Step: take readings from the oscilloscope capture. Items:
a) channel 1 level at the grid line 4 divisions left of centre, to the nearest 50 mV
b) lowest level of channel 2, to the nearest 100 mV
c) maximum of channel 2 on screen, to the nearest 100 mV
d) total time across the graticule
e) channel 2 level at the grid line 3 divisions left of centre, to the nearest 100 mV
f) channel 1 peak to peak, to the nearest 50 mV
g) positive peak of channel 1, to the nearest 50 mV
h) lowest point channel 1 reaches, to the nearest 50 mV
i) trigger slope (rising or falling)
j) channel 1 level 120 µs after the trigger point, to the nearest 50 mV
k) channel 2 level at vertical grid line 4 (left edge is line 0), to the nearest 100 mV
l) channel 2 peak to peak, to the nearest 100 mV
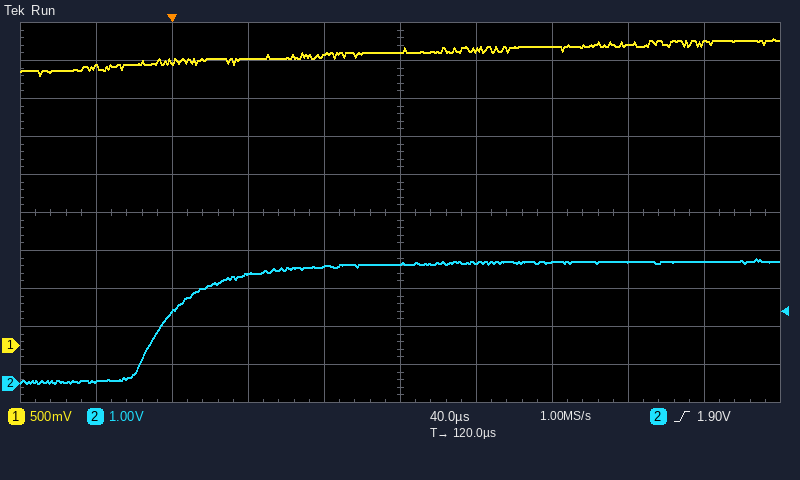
3.65 V
0.0 V
3.3 V
400 µs
1.9 V
500 mV
4.05 V
3.55 V
rising
3.85 V
3.1 V
3.3 V
